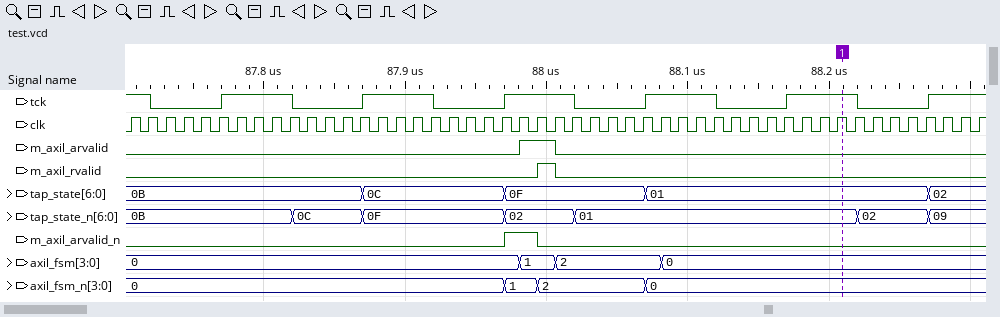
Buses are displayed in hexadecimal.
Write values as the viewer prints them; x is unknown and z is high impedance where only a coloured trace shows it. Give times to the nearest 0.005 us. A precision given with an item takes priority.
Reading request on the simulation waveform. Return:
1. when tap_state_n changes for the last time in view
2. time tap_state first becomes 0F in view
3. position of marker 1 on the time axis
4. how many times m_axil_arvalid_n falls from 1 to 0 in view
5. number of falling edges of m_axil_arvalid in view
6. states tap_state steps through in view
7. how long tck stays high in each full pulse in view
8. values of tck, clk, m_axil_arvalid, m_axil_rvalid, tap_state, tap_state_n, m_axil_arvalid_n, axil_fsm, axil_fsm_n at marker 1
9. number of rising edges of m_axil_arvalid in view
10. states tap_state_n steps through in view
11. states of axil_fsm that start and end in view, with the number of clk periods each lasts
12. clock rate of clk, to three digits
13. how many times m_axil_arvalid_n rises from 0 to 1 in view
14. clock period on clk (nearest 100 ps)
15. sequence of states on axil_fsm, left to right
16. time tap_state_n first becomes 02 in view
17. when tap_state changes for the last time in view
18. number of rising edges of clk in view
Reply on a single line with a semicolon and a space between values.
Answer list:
88.27 us; 87.97 us; 88.21 us; 1; 1; 0B, 0C, 0F, 01, 02; 0.05 us, 0.05 us, 0.05 us, 0.05 us, 0.05 us; tck=1, clk=1, m_axil_arvalid=0, m_axil_rvalid=0, tap_state=01, tap_state_n=01, m_axil_arvalid_n=0, axil_fsm=0, axil_fsm_n=0; 1; 0B, 0C, 0F, 02, 01, 02, 09; 1: 2, 2: 6; 80.0 MHz; 1; 12500 ps; 0, 1, 2, 0; 87.97 us; 88.27 us; 49
